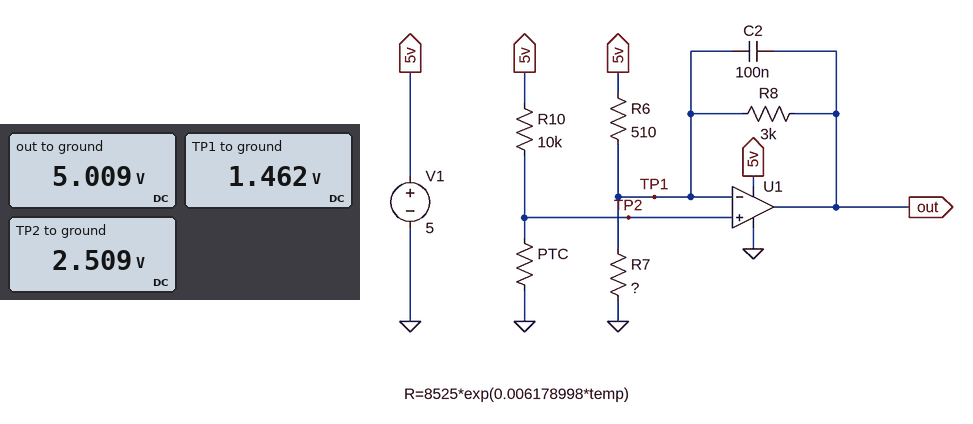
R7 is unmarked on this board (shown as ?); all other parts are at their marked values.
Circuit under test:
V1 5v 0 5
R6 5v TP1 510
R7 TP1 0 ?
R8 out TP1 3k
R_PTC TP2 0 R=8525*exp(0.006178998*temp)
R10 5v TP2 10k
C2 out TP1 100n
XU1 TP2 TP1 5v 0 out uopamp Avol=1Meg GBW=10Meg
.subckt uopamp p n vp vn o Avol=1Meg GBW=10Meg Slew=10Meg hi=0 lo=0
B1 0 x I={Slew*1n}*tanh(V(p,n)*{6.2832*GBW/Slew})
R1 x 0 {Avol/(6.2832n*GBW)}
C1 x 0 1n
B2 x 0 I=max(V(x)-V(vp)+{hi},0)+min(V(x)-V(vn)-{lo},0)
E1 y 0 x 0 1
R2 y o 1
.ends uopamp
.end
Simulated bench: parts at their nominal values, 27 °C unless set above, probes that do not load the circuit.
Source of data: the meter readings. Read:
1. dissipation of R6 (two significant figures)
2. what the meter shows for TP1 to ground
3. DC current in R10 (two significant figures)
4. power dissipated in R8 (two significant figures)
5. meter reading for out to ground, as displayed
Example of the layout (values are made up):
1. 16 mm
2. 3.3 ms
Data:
1. 25 mW
2. 1.462 V
3. 250 µA
4. 4.2 mW
5. 5.009 V
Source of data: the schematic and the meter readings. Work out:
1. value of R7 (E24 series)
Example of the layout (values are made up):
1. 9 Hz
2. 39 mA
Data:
1. 180 Ω
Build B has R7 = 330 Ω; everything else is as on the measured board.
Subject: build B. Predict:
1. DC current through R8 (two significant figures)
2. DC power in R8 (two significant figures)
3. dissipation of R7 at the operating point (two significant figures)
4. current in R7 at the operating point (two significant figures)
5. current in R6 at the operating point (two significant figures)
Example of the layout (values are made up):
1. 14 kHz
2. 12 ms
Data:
1. 950 µA
2. 2.7 mW
3. 14 mW
4. 6.5 mA
5. 5.6 mA
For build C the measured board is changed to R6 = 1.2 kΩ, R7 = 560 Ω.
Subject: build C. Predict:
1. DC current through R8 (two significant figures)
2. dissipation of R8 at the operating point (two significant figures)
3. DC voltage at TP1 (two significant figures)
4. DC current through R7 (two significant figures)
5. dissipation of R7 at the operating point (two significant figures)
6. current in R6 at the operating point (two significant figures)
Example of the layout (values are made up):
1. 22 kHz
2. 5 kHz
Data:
1. 1.0 mA
2. 3.1 mW
3. 2.0 V
4. 3.5 mA
5. 7.0 mW
6. 2.5 mA
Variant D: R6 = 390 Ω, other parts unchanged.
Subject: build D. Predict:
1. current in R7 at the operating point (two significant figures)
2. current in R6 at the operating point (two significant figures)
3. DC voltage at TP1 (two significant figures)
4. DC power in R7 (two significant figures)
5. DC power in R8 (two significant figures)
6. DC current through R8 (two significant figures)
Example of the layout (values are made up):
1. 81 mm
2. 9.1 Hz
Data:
1. 9.5 mA
2. 8.4 mA
3. 1.7 V
4. 16 mW
5. 3.6 mW
6. 1.1 mA
